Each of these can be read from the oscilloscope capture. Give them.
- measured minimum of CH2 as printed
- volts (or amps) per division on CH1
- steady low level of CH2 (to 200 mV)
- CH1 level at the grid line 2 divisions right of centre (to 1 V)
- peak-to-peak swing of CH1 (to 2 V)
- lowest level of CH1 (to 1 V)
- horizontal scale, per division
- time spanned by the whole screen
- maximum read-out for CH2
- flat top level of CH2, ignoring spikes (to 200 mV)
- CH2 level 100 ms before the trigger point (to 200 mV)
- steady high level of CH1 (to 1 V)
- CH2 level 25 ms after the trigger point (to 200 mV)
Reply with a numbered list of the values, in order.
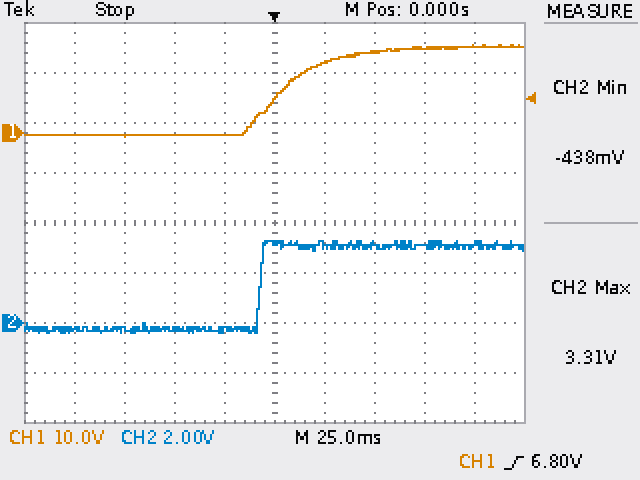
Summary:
1. -438 mV
2. 10 V
3. -200 mV
4. 16 V
5. 18 V
6. -1 V
7. 25 ms
8. 250 ms
9. 3.31 V
10. 3.2 V
11. -200 mV
12. 17 V
13. 3.2 V
